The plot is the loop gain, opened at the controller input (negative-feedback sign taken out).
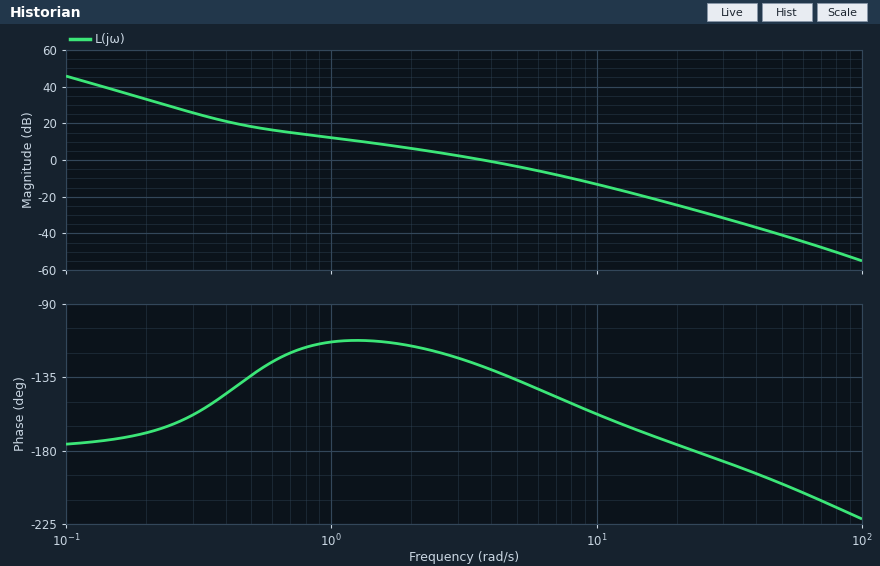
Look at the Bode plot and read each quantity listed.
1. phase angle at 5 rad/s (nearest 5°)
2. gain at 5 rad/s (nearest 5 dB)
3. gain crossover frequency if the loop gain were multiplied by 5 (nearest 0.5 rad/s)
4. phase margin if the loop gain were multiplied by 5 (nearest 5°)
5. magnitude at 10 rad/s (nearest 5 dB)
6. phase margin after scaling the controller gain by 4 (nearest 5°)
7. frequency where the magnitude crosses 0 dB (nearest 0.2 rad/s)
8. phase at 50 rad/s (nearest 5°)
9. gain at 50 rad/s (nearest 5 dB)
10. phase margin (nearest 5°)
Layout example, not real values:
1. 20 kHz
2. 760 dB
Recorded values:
1. -135°
2. -5 dB
3. 10.5 rad/s
4. 20°
5. -15 dB
6. 25°
7. 3.8 rad/s
8. -200°
9. -40 dB
10. 50°
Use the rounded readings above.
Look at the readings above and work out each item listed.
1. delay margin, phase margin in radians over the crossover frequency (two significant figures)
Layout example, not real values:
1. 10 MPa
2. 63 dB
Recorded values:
1. 0.23 s
